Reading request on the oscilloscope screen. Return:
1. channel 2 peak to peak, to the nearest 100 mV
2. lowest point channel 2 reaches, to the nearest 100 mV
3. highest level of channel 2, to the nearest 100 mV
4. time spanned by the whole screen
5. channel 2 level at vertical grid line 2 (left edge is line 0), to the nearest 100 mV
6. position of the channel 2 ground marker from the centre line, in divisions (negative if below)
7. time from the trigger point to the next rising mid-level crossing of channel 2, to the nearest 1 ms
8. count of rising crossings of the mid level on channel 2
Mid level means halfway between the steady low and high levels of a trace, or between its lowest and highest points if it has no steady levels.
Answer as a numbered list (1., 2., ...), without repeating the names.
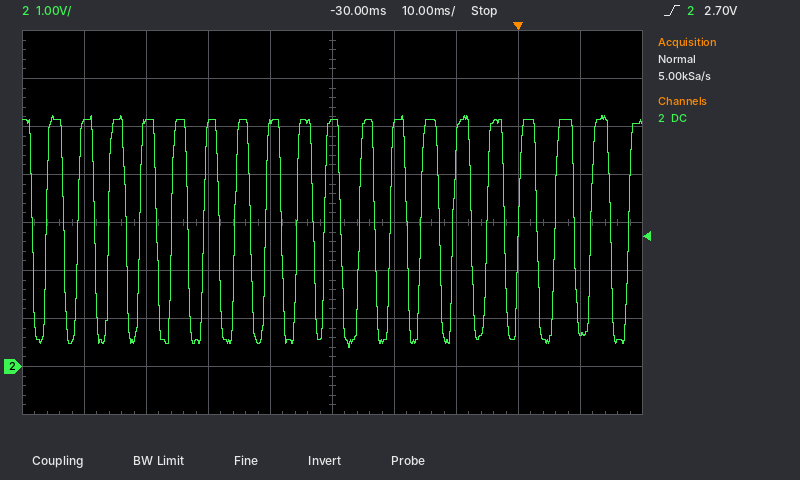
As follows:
1. 4.8 V
2. 400 mV
3. 5.2 V
4. 100 ms
5. 5.1 V
6. -3.0 div
7. 6 ms
8. 19
